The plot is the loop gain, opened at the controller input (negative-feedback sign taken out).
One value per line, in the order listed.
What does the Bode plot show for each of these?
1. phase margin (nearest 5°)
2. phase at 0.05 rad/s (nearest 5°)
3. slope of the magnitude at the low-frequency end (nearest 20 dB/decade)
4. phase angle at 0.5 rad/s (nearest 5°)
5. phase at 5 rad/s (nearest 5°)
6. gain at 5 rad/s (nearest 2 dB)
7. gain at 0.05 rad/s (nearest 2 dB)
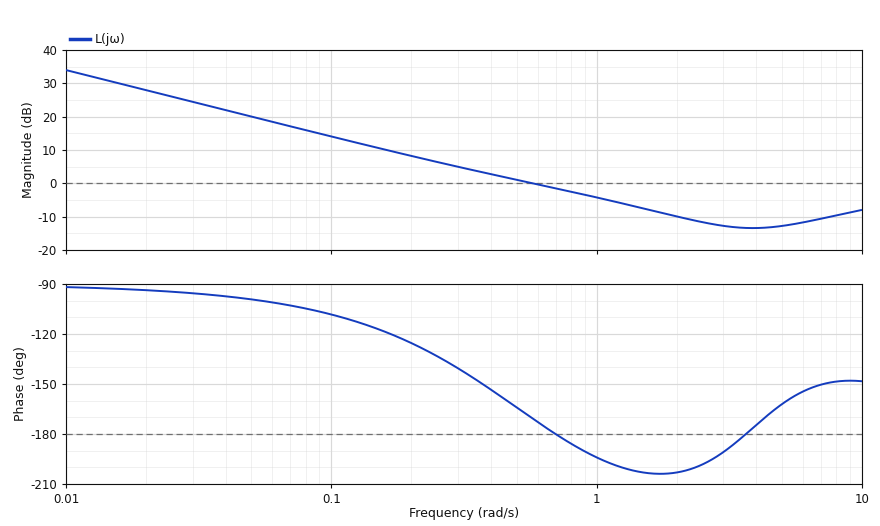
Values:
10°
-100°
-20 dB/decade
-165°
-160°
-12 dB
20 dB
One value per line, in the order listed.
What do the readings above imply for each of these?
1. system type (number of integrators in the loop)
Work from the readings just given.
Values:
1
